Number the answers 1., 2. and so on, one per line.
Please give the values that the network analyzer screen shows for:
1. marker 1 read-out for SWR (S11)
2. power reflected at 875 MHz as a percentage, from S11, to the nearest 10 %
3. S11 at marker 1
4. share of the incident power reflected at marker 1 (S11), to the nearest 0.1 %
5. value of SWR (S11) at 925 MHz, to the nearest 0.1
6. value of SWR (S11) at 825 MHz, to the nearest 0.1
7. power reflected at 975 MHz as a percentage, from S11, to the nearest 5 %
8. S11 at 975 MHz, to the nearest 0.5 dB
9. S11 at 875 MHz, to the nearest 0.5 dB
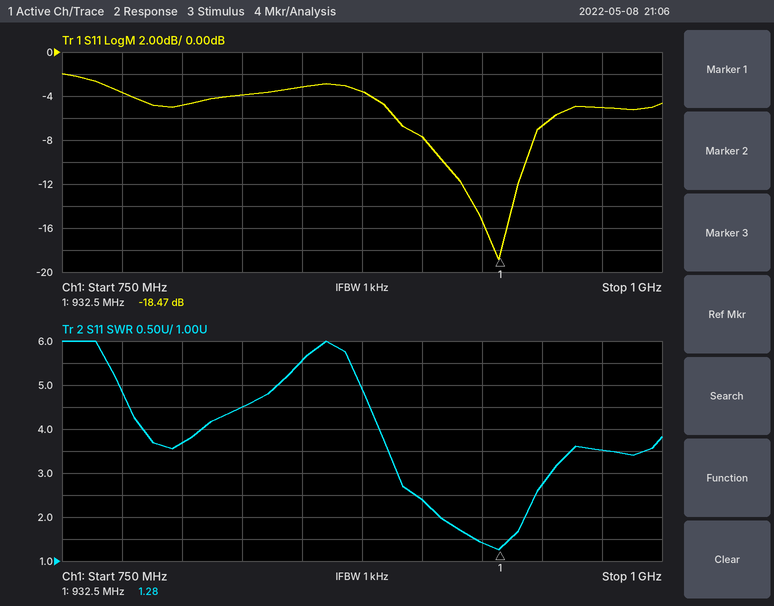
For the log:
1. 1.28
2. 40 %
3. -18.47 dB
4. 1.4 %
5. 1.4
6. 4.5
7. 30 %
8. -5.0 dB
9. -3.5 dB
